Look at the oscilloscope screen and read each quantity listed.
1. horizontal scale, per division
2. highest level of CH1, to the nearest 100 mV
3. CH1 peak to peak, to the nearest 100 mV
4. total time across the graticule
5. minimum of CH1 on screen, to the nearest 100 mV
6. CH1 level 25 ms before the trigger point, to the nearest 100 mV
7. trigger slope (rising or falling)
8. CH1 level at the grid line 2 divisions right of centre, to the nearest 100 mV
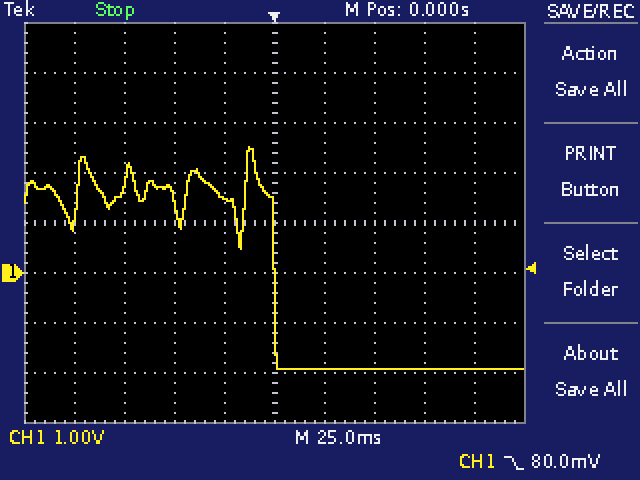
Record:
25 ms
2.5 V
4.4 V
250 ms
-1.9 V
1.5 V
falling
-1.9 V
